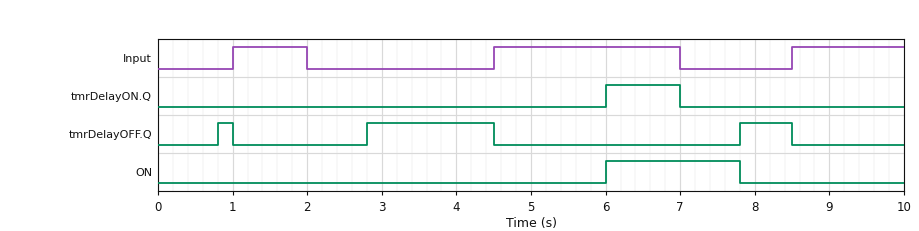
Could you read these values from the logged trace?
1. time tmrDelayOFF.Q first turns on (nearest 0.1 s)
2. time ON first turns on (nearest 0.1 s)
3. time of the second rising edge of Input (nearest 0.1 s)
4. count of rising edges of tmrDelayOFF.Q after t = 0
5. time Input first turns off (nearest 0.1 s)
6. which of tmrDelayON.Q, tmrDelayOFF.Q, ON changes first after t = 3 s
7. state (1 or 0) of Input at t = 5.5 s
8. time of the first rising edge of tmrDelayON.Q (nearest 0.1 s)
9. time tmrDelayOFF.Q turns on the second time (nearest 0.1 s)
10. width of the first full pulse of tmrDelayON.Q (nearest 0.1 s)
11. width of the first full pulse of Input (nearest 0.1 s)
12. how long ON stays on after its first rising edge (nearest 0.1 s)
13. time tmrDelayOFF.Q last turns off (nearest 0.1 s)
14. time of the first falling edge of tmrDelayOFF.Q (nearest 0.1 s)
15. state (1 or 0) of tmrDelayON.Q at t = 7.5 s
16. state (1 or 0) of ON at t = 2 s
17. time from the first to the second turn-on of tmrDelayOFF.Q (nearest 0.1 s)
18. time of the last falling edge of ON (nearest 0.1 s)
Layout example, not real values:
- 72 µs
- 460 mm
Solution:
- 0.8 s
- 6.0 s
- 4.5 s
- 3
- 2.0 s
- tmrDelayOFF.Q
- 1
- 6.0 s
- 2.8 s
- 1.0 s
- 1.0 s
- 1.8 s
- 8.5 s
- 1.0 s
- 0
- 0
- 2.0 s
- 7.8 s
